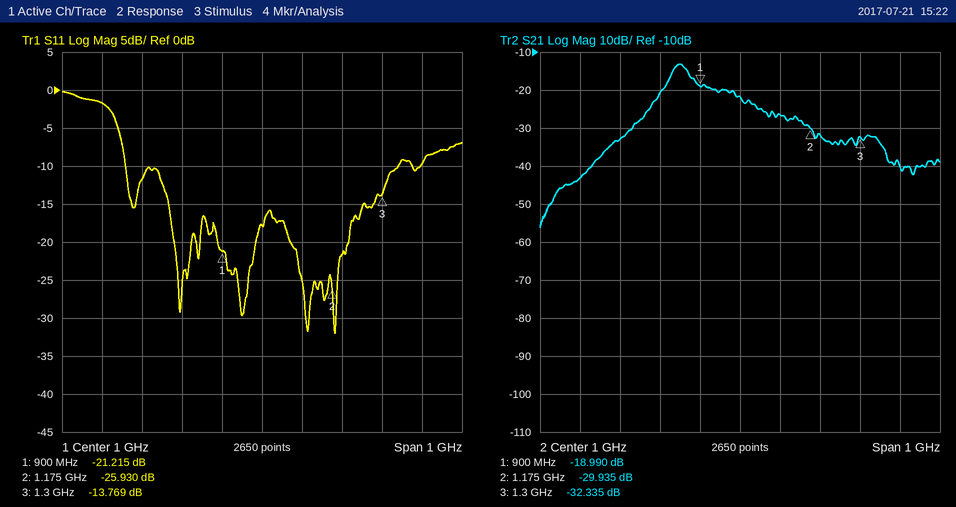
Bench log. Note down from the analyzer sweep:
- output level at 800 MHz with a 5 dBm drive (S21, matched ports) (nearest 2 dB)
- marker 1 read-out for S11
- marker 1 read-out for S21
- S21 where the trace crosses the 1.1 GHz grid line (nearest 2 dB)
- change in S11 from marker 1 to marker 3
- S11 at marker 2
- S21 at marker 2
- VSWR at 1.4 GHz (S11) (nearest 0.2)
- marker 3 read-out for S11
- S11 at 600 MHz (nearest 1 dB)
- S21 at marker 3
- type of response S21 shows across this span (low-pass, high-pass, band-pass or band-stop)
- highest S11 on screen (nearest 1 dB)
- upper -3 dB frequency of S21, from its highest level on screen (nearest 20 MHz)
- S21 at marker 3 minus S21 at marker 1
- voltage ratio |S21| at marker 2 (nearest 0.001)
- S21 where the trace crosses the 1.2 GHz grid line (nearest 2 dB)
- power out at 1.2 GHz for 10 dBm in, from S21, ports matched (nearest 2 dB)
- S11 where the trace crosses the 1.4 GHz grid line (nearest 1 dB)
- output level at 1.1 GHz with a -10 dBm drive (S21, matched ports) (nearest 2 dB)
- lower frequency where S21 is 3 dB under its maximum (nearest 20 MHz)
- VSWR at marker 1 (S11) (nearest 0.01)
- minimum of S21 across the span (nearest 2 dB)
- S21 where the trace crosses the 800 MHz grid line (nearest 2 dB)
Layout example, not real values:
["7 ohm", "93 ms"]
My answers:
["-16 dBm", "-21.215 dB", "-18.990 dB", "-26 dB", "7.446 dB", "-25.930 dB", "-29.935 dB", "2.0", "-13.769 dB", "-2 dB", "-32.335 dB", "band-pass", "0 dB", "880 MHz", "-13.345 dB", "0.032", "-32 dB", "-22 dBm", "-10 dB", "-36 dBm", "820 MHz", "1.19", "-56 dB", "-20 dB"]
